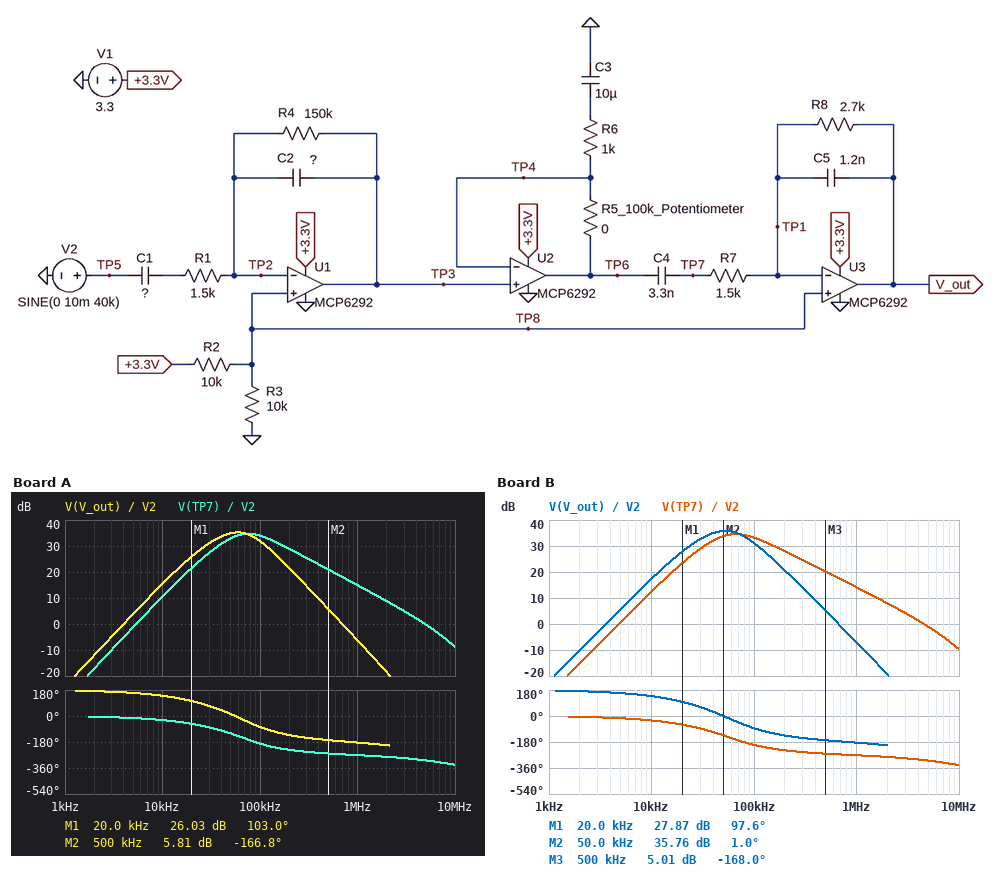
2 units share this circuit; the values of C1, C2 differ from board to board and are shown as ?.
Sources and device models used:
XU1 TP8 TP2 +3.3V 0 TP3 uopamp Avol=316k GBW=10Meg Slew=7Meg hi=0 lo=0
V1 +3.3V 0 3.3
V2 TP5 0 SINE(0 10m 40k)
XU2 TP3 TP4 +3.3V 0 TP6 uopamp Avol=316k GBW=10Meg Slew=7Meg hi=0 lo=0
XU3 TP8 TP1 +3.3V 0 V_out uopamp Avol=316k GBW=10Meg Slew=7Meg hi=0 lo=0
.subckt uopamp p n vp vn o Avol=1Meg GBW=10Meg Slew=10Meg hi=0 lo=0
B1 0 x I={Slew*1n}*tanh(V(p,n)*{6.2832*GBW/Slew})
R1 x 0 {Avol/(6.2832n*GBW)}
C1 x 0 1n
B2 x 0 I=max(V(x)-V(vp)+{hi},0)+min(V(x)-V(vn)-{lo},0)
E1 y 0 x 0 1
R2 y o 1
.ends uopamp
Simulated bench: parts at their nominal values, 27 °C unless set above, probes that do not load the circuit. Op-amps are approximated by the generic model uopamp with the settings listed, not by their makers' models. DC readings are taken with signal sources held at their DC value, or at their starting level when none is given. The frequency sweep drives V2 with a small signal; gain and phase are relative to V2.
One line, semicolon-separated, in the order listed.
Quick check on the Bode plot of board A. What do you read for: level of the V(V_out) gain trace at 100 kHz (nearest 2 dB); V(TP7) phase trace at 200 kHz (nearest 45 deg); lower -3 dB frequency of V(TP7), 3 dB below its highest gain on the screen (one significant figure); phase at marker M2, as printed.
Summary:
32 dB; -225 deg; 40 kHz; -166.8 deg
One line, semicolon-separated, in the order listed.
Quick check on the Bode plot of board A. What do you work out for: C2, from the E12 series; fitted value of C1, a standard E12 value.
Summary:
8.2 pF; 1.2 nF
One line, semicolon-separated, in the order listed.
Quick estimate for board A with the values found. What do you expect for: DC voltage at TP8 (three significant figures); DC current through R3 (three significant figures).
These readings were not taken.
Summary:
1.65 V; 165 µA
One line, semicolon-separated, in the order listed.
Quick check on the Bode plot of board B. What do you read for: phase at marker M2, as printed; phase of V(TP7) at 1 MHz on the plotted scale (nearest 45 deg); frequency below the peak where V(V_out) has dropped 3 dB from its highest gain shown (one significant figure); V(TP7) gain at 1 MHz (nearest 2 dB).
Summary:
1.0 deg; -270 deg; 30 kHz; 14 dB
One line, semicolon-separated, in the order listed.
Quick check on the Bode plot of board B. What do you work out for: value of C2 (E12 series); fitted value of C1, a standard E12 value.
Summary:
10 pF; 1.5 nF
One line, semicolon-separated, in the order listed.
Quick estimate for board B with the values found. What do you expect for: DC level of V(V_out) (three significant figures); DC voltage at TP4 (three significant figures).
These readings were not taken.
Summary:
1.65 V; 1.65 V
